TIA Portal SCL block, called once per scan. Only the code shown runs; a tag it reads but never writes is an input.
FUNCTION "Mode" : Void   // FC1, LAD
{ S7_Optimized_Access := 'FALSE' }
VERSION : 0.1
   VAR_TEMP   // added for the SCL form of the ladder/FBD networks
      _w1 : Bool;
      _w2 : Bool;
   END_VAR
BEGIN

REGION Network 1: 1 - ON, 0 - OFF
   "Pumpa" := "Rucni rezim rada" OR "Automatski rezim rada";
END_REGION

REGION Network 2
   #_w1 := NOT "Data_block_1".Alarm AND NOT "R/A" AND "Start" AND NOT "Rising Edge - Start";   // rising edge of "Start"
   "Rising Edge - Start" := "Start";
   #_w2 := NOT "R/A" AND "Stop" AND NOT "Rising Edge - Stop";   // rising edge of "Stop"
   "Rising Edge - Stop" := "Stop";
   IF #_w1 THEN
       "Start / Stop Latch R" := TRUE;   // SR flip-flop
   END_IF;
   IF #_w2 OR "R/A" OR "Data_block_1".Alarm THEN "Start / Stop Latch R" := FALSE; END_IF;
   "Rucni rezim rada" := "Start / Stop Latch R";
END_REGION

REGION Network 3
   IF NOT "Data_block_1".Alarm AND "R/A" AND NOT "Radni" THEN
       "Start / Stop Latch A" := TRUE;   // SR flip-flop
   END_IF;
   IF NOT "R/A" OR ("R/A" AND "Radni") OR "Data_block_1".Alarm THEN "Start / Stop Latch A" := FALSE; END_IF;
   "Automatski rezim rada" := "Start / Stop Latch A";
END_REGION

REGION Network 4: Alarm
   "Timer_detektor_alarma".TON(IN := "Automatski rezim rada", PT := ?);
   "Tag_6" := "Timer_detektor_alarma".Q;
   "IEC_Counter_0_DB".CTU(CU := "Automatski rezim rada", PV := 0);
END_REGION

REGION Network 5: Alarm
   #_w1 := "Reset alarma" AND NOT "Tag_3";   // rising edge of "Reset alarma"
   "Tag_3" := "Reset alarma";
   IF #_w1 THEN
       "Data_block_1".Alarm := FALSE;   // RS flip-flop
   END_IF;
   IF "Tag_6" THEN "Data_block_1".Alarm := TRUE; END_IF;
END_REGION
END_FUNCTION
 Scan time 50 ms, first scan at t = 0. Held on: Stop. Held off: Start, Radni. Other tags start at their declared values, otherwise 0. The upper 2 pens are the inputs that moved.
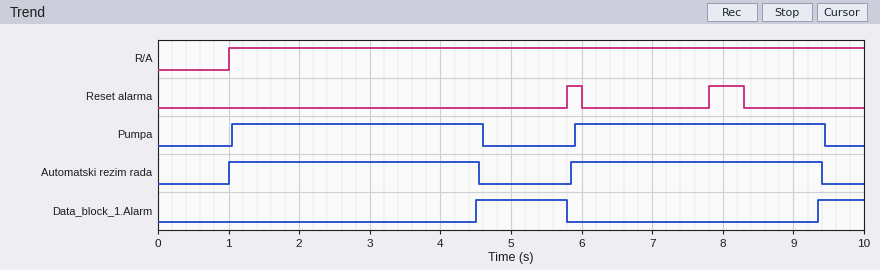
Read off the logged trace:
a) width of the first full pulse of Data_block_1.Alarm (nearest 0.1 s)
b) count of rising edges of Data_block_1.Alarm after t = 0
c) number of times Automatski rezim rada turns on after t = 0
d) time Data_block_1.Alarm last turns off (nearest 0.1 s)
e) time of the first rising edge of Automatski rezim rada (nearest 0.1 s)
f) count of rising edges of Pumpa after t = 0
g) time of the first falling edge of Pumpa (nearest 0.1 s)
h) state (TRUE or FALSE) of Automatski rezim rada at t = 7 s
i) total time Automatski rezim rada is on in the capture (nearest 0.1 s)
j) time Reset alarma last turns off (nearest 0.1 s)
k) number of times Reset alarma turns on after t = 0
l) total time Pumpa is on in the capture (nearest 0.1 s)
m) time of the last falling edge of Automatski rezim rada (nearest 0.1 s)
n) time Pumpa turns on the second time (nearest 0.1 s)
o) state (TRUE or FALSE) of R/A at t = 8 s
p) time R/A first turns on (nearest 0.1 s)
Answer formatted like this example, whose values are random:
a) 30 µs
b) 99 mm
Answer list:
a) 1.3 s
b) 2
c) 2
d) 5.8 s
e) 1.0 s
f) 2
g) 4.6 s
h) TRUE
i) 7.1 s
j) 8.3 s
k) 2
l) 7.1 s
m) 9.4 s
n) 5.9 s
o) TRUE
p) 1.0 s
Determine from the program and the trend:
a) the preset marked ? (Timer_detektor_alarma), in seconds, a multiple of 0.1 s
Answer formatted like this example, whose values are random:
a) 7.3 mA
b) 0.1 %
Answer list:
a) 3.5 s
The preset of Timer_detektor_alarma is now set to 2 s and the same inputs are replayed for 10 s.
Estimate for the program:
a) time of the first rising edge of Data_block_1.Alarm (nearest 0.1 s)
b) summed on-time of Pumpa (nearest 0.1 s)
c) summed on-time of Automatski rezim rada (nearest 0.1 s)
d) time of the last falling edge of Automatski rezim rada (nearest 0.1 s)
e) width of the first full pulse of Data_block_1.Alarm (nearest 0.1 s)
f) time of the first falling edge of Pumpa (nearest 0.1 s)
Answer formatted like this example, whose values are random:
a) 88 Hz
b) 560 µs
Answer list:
a) 3.0 s
b) 4.1 s
c) 4.1 s
d) 7.9 s
e) 2.8 s
f) 3.1 s
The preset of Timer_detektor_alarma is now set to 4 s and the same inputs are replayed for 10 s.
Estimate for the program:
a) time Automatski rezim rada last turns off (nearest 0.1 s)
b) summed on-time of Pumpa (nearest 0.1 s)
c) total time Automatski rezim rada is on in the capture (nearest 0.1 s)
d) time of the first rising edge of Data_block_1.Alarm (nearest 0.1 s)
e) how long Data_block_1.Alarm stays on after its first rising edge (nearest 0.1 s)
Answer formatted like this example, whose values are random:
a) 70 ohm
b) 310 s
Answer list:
a) 9.9 s
b) 8.1 s
c) 8.1 s
d) 5.0 s
e) 0.8 s
